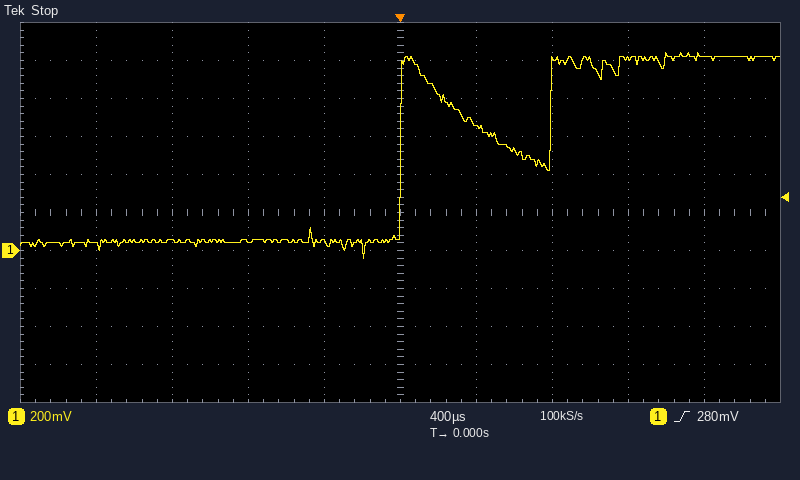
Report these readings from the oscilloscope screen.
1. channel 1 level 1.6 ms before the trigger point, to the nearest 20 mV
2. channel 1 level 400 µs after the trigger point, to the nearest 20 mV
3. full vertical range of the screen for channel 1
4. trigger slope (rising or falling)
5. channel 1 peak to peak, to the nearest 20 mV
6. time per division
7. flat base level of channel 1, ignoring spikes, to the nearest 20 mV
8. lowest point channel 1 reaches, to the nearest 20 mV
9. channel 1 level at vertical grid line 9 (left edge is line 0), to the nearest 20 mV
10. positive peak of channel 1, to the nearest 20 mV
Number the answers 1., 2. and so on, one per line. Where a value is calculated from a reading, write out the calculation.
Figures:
1. 20 mV
2. 660 mV
3. 2 V
4. rising
5. 1.04 V − (-40 mV) = 1.08 V
6. 400 µs
7. 40 mV
8. -40 mV
9. 1.02 V
10. 1.04 V
